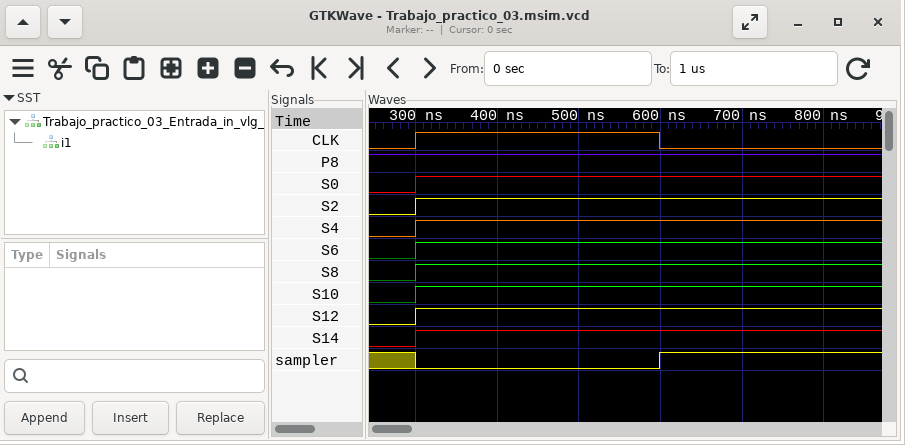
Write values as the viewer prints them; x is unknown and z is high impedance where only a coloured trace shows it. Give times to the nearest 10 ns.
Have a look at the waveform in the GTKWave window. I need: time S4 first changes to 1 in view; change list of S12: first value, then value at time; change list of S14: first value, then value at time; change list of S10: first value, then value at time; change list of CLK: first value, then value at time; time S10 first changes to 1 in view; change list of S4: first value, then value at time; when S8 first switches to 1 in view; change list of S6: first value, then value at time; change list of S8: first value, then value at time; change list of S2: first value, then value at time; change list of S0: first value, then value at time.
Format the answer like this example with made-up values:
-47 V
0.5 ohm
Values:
300 ns
0, 1 at 300 ns
0, 1 at 300 ns
0, 1 at 300 ns
0, 1 at 300 ns, 0 at 600 ns
300 ns
0, 1 at 300 ns
300 ns
0, 1 at 300 ns
0, 1 at 300 ns
0, 1 at 300 ns
0, 1 at 300 ns
